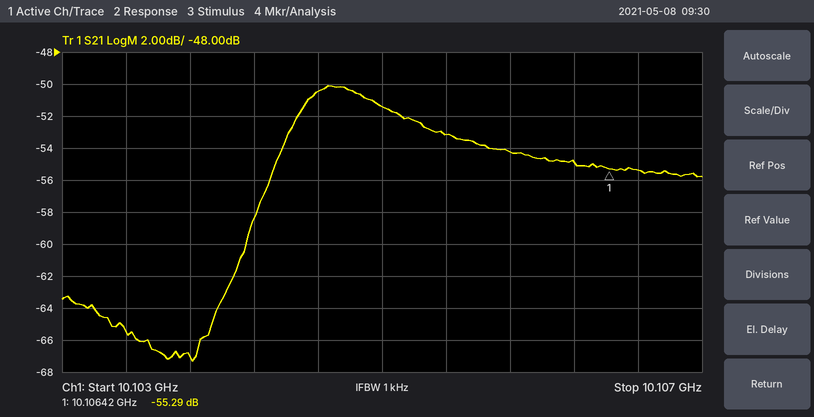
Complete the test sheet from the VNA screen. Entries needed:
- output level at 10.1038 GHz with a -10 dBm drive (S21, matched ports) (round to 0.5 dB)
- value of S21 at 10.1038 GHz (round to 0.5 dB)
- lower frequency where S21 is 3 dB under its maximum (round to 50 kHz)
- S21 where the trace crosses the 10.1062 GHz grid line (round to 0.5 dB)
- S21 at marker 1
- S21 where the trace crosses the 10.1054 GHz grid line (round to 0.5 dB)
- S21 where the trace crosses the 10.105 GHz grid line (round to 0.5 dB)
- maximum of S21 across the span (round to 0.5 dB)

-77.0 dBm
-67.0 dB
10.10440 GHz
-55.0 dB
-55.29 dB
-53.0 dB
-51.5 dB
-50.0 dB
